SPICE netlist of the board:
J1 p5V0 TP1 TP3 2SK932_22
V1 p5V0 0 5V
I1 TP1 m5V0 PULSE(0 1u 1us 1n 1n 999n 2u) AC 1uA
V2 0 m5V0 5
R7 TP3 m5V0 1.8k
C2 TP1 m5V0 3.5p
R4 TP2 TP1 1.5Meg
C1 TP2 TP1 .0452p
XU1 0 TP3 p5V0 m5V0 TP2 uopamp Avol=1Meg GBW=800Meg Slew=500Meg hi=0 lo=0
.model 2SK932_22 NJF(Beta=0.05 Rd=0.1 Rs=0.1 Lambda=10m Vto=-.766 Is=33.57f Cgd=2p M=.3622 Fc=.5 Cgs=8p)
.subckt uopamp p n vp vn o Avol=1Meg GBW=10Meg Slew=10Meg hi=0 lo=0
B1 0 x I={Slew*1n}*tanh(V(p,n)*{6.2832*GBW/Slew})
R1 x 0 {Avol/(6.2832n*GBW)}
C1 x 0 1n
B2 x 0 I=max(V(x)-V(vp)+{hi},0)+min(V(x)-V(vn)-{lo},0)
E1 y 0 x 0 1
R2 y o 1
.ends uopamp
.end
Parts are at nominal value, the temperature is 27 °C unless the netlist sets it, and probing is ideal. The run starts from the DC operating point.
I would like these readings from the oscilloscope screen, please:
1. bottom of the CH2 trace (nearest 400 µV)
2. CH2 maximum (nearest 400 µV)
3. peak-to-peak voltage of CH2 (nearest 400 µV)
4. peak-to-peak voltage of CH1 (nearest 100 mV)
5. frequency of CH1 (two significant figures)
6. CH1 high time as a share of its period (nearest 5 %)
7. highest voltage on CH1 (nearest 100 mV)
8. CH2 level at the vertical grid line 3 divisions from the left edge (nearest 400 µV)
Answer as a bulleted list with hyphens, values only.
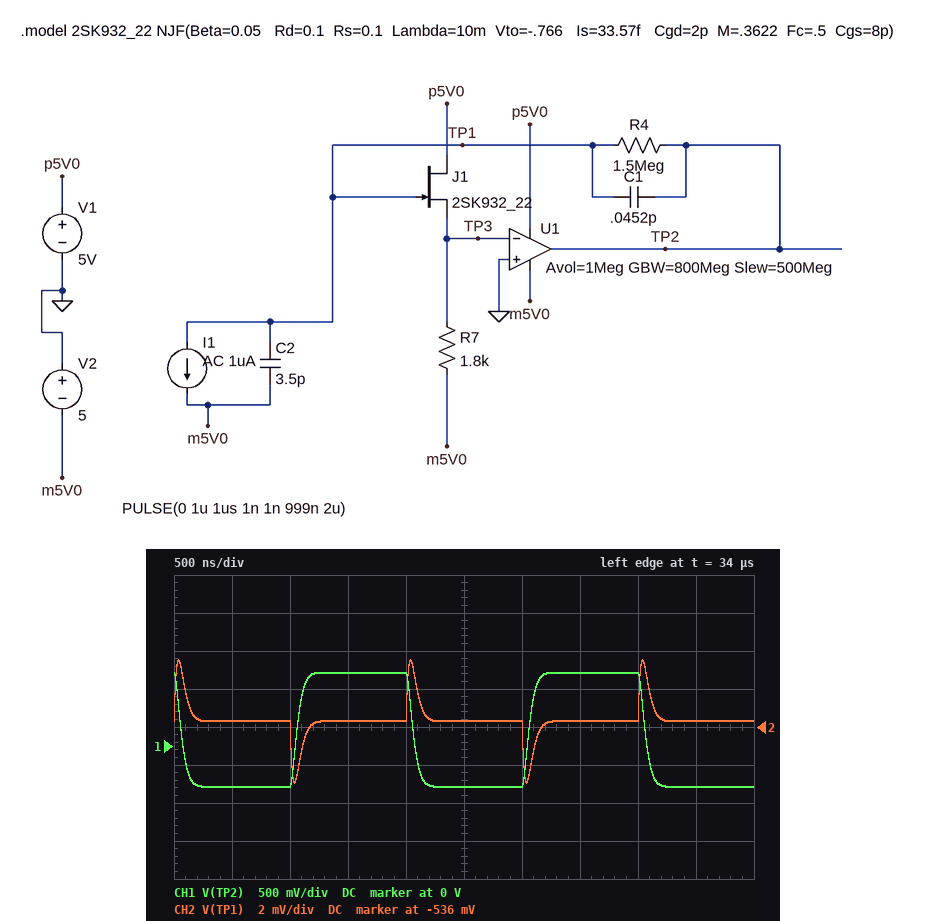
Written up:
- -538.8 mV
- -532.4 mV
- 6.4 mV
- 1.5 V
- 500 kHz
- 50 %
- 1.0 V
- -535.6 mV
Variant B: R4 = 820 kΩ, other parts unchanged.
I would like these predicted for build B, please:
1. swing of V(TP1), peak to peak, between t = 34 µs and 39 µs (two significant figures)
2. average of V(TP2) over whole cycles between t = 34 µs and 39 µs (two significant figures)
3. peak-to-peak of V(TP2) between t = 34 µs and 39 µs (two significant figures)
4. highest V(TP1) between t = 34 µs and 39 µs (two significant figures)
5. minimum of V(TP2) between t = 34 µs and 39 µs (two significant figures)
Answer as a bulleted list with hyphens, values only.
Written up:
- 5.7 mV
- -130 mV
- 910 mV
- -530 mV
- -580 mV
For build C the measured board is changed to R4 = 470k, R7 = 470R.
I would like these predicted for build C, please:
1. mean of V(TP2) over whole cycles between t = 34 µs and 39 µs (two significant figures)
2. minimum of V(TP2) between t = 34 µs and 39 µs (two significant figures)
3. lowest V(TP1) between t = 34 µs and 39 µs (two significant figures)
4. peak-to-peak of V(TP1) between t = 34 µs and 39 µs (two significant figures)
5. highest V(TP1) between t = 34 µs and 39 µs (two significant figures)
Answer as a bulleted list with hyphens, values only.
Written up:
- -80 mV
- -390 mV
- -320 mV
- 5.0 mV
- -310 mV
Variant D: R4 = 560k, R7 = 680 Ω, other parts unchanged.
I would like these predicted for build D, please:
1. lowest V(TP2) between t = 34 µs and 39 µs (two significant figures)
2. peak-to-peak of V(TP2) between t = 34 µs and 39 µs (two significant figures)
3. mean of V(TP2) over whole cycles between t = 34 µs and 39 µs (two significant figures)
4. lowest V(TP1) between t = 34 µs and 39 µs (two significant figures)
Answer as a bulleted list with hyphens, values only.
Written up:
- -460 mV
- 700 mV
- -110 mV
- -390 mV
